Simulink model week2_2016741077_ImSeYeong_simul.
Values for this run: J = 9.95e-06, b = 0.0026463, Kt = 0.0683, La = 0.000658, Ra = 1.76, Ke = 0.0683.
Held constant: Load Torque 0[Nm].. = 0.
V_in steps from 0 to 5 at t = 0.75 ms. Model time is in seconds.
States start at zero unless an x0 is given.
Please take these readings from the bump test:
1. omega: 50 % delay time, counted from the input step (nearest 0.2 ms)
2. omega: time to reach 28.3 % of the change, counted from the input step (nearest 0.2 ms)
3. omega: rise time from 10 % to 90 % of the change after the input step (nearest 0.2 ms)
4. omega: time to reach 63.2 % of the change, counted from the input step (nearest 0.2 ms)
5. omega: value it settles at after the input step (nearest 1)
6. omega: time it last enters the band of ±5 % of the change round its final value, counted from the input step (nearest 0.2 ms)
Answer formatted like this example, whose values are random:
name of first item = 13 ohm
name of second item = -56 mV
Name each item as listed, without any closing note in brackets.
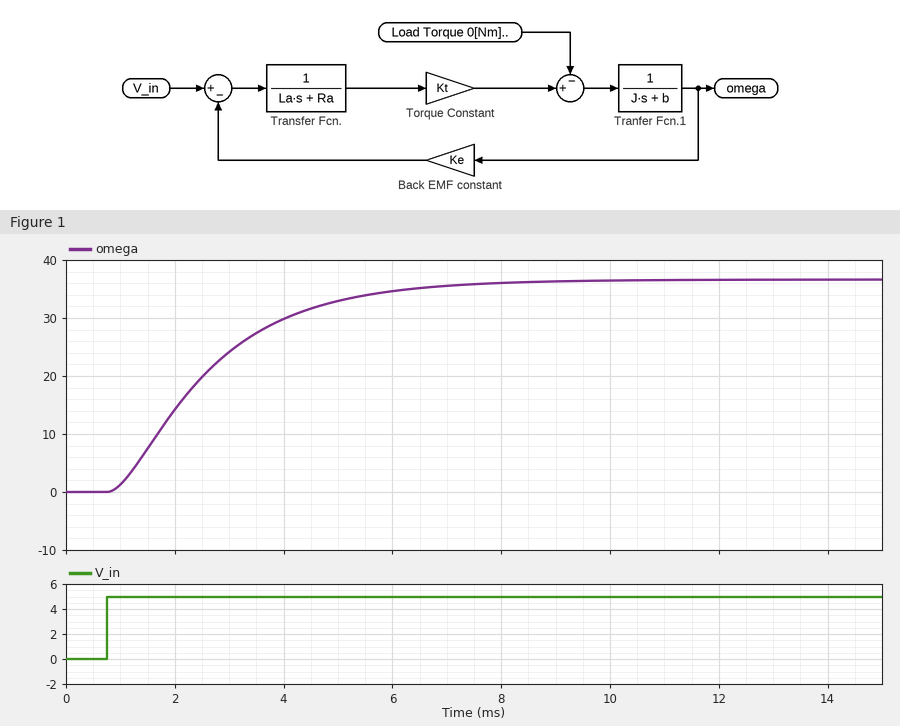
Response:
omega: 50 % delay time, counted from the input step = 1.6 ms
omega: time to reach 28.3 % of the change, counted from the input step = 1.0 ms
omega: rise time from 10 % to 90 % of the change after the input step = 3.8 ms
omega: time to reach 63.2 % of the change, counted from the input step = 2.2 ms
omega: value it settles at after the input step = 37
omega: time it last enters the band of ±5 % of the change round its final value, counted from the input step = 5.4 ms
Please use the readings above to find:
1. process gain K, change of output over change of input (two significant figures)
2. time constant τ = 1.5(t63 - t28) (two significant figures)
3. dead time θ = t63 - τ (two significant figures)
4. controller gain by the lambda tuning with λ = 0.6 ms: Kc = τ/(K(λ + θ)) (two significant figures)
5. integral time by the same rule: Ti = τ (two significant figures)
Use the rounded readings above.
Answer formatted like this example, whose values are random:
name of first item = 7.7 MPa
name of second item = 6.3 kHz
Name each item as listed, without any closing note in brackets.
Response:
process gain K, change of output over change of input = 7.4
time constant τ = 1.5(t63 - t28) = 1.8 ms
dead time θ = t63 - τ = 0.40 ms
controller gain by the lambda tuning with λ = 0.6 ms: Kc = τ/(K(λ + θ)) = 0.24
integral time by the same rule: Ti = τ = 1.8 ms
